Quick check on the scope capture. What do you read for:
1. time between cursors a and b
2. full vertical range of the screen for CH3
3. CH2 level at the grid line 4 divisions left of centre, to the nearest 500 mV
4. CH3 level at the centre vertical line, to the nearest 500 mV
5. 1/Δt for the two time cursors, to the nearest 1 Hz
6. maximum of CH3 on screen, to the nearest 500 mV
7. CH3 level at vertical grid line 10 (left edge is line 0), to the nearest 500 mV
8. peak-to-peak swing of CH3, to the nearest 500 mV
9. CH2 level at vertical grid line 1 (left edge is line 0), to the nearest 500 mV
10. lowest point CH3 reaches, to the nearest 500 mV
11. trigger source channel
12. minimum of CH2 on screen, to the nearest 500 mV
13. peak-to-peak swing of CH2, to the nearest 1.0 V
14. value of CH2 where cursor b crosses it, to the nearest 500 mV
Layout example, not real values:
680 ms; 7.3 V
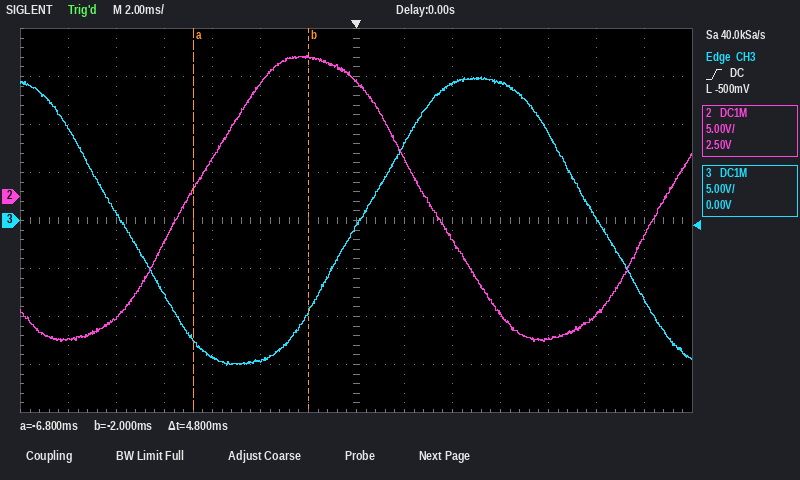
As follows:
4.8 ms; 40 V; -5.0 V; -500 mV; 208 Hz; 15.0 V; 14.5 V; 30.0 V; -15.0 V; -15.0 V; CH3; -15.0 V; 30.0 V; 14.5 V
